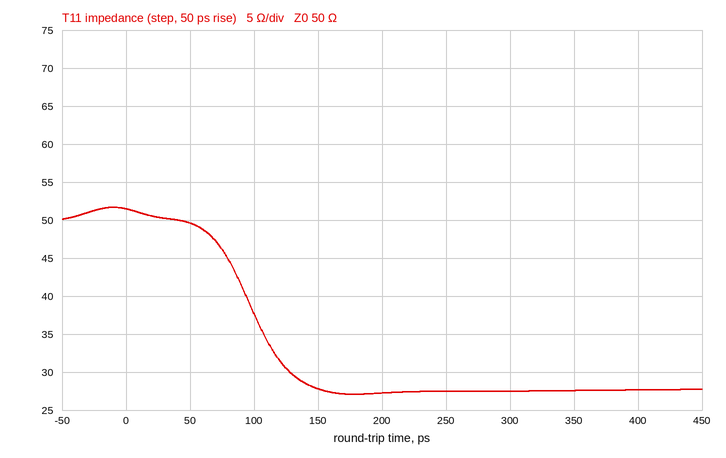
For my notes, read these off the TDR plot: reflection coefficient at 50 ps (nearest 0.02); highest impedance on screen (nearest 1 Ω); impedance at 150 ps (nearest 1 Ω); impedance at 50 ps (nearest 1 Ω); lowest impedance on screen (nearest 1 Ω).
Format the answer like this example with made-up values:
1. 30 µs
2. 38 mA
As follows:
1. 0.00
2. 52 Ω
3. 28 Ω
4. 50 Ω
5. 27 Ω
